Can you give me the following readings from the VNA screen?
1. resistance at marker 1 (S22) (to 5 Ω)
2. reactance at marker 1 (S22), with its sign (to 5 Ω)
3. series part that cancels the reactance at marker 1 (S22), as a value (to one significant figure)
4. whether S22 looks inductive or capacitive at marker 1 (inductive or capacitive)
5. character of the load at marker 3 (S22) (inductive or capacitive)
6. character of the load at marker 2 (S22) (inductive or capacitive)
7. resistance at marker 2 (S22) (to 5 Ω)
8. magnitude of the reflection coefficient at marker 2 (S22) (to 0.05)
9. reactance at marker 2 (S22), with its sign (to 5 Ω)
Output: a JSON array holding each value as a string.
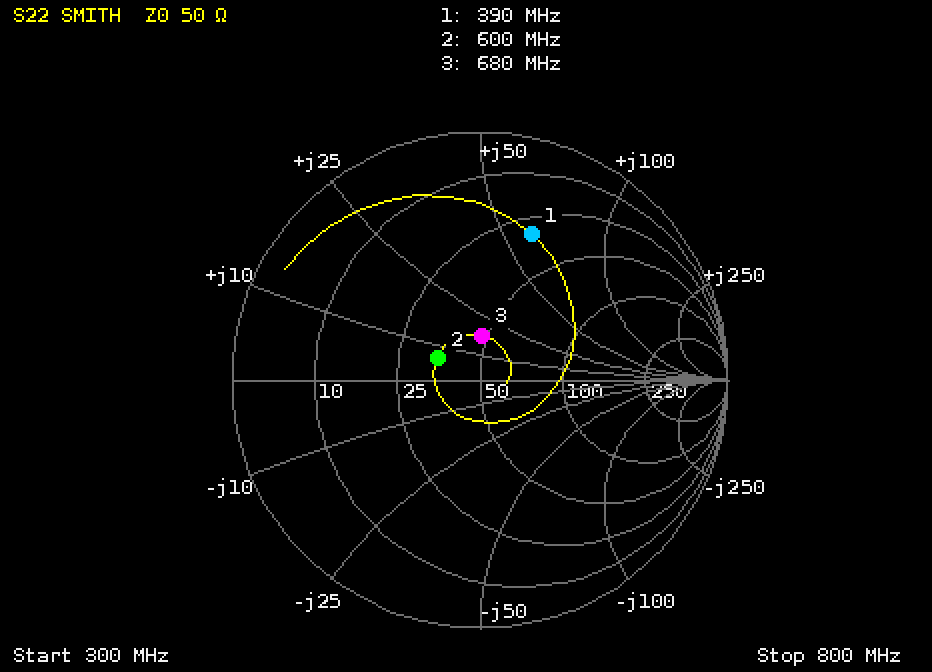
["30 Ω", "+60 Ω", "7 pF", "inductive", "inductive", "inductive", "35 Ω", "0.20", "+5 Ω"]
